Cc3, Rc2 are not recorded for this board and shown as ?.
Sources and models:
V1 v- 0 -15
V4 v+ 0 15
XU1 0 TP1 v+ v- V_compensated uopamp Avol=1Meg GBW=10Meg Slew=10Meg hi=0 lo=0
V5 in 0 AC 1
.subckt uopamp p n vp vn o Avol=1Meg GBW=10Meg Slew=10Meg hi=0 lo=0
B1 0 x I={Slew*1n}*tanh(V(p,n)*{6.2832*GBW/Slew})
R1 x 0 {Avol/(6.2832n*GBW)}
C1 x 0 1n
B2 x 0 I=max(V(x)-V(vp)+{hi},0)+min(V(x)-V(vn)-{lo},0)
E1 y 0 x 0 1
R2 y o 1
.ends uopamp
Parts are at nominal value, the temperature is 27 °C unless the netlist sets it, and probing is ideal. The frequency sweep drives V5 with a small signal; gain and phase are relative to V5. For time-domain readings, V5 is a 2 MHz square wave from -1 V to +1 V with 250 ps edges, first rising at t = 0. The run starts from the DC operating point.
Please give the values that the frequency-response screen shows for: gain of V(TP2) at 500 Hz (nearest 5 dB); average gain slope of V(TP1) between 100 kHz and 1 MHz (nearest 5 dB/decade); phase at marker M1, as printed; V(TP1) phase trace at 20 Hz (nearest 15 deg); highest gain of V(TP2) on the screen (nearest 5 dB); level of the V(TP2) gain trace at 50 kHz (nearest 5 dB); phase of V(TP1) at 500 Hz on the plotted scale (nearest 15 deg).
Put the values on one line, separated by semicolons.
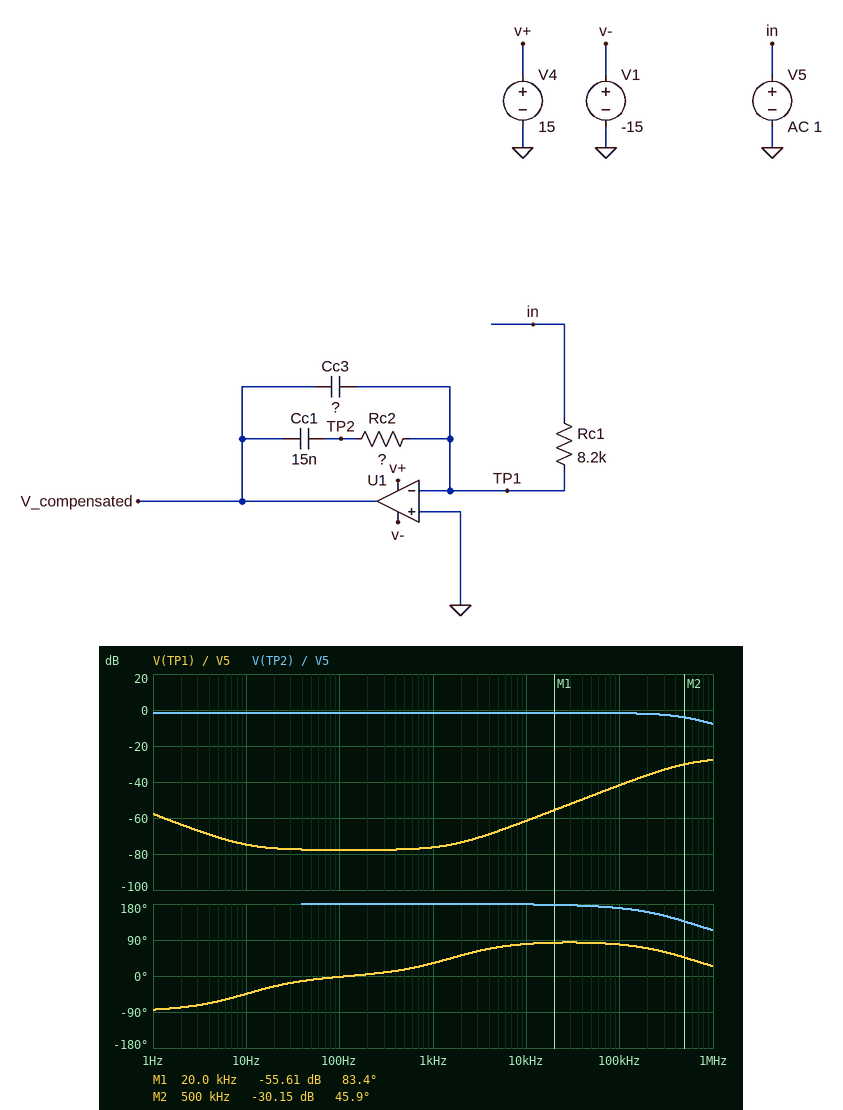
0 dB; 15 dB/decade; 83.4 deg; -30 deg; 0 dB; 0 dB; 15 deg
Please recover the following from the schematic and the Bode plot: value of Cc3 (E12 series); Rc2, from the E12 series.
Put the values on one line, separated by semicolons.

39 pF; 6.8 kΩ
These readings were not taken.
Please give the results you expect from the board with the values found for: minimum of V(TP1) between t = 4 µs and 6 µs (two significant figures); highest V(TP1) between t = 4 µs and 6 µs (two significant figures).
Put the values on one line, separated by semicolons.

-850 mV; -220 mV
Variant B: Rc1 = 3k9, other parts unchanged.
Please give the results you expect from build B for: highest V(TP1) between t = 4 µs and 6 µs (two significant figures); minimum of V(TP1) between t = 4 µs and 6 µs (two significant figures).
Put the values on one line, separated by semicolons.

36 mV; -890 mV
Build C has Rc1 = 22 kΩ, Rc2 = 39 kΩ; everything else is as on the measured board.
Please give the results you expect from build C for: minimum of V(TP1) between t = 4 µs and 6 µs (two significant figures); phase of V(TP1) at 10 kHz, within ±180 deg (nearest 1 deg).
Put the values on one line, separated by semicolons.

-500 mV; 83 deg
